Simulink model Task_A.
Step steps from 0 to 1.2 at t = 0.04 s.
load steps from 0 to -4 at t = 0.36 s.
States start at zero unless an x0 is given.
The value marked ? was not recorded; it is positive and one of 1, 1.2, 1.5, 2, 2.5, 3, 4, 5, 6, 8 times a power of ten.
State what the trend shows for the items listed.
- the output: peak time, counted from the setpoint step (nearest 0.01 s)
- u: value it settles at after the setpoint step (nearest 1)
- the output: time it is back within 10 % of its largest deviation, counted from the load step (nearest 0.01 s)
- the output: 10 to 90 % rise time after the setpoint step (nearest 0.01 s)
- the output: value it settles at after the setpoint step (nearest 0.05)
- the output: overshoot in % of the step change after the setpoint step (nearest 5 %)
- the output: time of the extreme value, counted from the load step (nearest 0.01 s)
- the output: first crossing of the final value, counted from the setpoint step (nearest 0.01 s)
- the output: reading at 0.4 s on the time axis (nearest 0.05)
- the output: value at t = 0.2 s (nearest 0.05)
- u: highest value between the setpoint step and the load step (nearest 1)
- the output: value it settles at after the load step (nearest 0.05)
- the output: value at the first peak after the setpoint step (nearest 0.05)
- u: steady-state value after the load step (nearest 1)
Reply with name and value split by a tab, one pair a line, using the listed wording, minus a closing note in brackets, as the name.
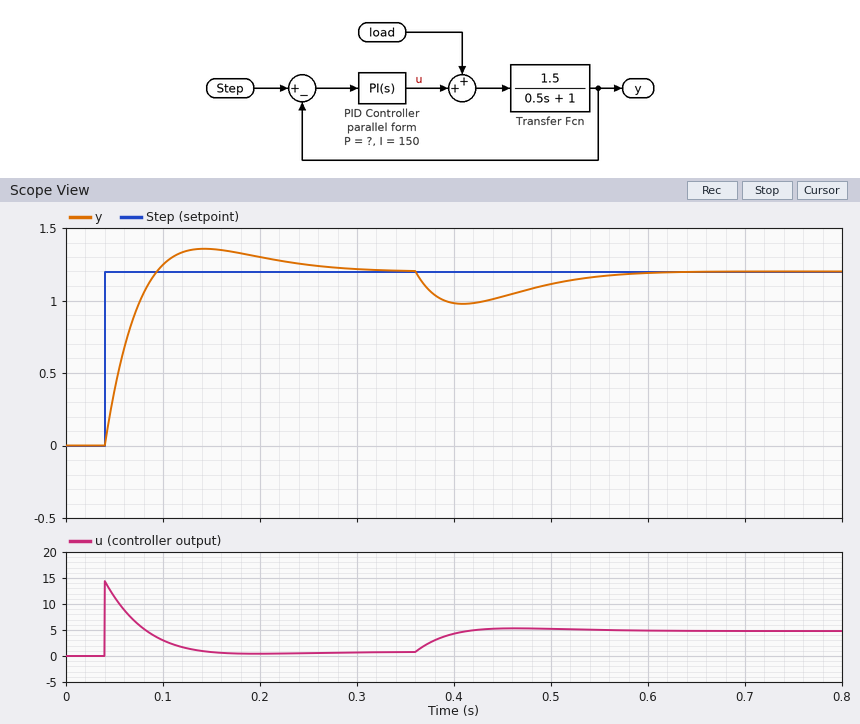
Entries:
the output: peak time, counted from the setpoint step	0.10 s
u: value it settles at after the setpoint step	1
the output: time it is back within 10 % of its largest deviation, counted from the load step	0.21 s
the output: 10 to 90 % rise time after the setpoint step	0.04 s
the output: value it settles at after the setpoint step	1.20
the output: overshoot in % of the step change after the setpoint step	15 %
the output: time of the extreme value, counted from the load step	0.05 s
the output: first crossing of the final value, counted from the setpoint step	0.05 s
the output: reading at 0.4 s on the time axis	1.00
the output: value at t = 0.2 s	1.30
u: highest value between the setpoint step and the load step	14
the output: value it settles at after the load step	1.20
the output: value at the first peak after the setpoint step	1.35
u: steady-state value after the load step	5
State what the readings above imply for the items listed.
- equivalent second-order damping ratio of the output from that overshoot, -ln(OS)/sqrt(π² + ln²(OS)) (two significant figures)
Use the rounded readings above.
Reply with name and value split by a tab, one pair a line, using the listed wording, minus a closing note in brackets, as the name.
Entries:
equivalent second-order damping ratio of the output from that overshoot, -ln(OS)/sqrt(π² + ln²(OS))	0.52
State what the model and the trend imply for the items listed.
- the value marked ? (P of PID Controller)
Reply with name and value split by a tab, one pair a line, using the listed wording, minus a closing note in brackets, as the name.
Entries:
the value marked ?	12
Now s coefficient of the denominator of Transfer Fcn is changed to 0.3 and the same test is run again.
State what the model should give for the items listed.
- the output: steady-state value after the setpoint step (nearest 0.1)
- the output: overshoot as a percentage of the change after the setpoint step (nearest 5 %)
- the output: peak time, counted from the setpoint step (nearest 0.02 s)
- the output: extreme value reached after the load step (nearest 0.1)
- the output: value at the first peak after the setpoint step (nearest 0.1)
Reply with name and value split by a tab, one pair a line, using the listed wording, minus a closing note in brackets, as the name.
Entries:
the output: steady-state value after the setpoint step	1.2
the output: overshoot as a percentage of the change after the setpoint step	10 %
the output: peak time, counted from the setpoint step	0.08 s
the output: extreme value reached after the load step	1.0
the output: value at the first peak after the setpoint step	1.3
